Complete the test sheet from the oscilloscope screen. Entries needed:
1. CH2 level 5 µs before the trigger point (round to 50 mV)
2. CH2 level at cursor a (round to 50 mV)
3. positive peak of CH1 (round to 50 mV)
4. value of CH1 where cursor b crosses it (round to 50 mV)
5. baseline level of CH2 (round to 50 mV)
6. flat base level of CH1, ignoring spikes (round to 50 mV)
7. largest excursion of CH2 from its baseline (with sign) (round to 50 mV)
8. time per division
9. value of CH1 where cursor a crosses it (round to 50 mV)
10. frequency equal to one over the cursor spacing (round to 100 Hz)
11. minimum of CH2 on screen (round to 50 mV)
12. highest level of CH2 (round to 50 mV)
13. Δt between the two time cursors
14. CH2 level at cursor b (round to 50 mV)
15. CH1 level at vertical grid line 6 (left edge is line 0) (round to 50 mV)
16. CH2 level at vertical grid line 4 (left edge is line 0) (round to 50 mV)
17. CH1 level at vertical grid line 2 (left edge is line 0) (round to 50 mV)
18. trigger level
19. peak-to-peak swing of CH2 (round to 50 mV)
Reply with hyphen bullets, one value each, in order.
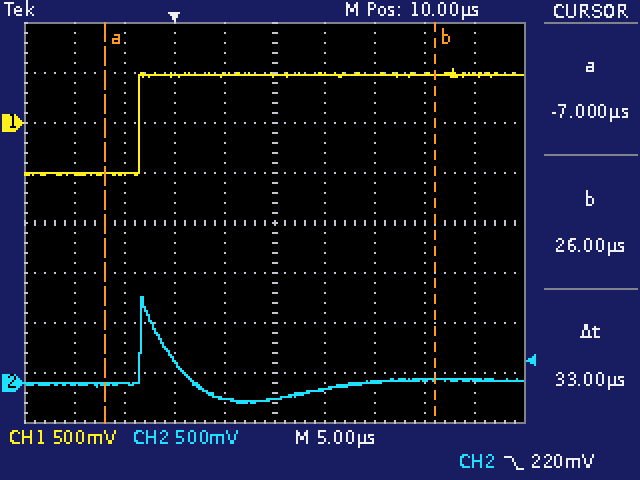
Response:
- 0 mV
- 0 mV
- 550 mV
- 500 mV
- 0 mV
- -500 mV
- +850 mV
- 5 µs
- -500 mV
- 30.3 kHz
- -200 mV
- 850 mV
- 33 µs
- 50 mV
- 500 mV
- -150 mV
- -500 mV
- 220 mV
- 1.05 V
